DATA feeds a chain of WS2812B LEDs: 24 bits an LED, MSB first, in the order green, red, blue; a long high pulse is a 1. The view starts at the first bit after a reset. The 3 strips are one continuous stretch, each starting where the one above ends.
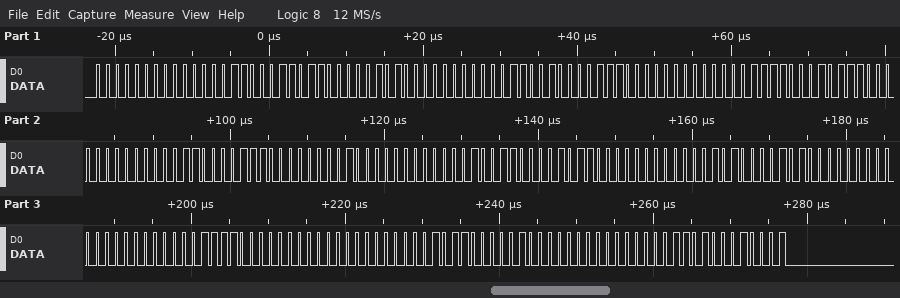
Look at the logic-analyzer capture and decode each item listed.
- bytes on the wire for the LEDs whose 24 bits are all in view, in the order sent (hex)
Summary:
00 03 1B 05 00 19 0E 00 0F 17 00 06 1C 02 00 13 0B 00 0A 14 00 00 1E 00 00 16 08 00 0D 11
